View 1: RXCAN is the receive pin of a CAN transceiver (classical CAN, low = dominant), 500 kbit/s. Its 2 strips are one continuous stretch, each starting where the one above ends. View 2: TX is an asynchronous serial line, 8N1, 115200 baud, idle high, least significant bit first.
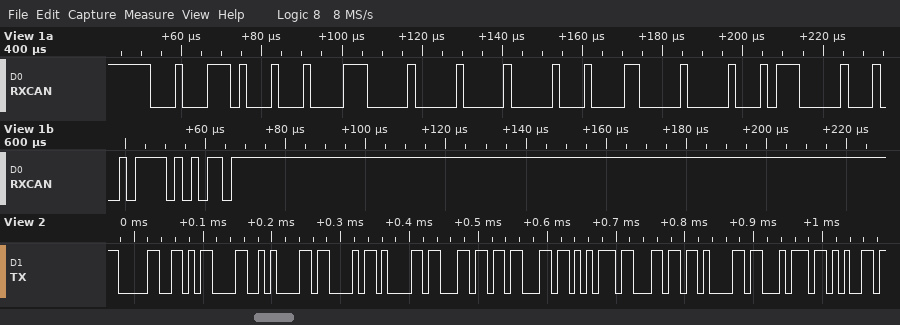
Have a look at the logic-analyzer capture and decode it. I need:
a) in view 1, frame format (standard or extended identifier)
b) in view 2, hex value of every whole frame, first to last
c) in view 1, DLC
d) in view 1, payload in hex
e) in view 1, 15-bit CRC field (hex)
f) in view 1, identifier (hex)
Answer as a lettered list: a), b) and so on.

a) standard
b) 30 0D 0A 43 61 6C 63 75 6C 61 74 65
c) 8
d) 87 00 00 01 0C 00 17 00
e) 0x4BD5
f) 0x11D
